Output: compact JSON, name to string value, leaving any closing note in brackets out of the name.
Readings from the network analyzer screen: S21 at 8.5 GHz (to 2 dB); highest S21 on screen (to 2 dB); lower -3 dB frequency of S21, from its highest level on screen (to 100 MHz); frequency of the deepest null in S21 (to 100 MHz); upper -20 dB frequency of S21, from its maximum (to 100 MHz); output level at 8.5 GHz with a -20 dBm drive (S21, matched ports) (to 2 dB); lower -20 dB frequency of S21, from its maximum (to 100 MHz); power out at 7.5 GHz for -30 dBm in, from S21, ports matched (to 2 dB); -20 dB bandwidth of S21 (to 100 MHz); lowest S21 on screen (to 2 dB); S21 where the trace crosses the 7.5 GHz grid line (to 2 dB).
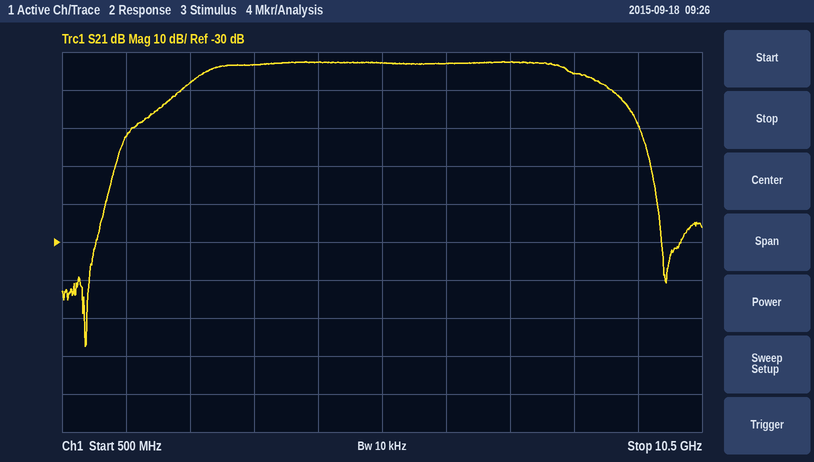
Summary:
{"S21 at 8.5 GHz": "14 dB", "highest S21 on screen": "18 dB", "lower -3 dB frequency of S21, from its highest level on screen": "2.7 GHz", "frequency of the deepest null in S21": "900 MHz", "upper -20 dB frequency of S21, from its maximum": "9.6 GHz", "output level at 8.5 GHz with a -20 dBm drive (S21, matched ports)": "-6 dBm", "lower -20 dB frequency of S21, from its maximum": "1.5 GHz", "power out at 7.5 GHz for -30 dBm in, from S21, ports matched": "-12 dBm", "-20 dB bandwidth of S21": "8.1 GHz", "lowest S21 on screen": "-58 dB", "S21 where the trace crosses the 7.5 GHz grid line": "18 dB"}
